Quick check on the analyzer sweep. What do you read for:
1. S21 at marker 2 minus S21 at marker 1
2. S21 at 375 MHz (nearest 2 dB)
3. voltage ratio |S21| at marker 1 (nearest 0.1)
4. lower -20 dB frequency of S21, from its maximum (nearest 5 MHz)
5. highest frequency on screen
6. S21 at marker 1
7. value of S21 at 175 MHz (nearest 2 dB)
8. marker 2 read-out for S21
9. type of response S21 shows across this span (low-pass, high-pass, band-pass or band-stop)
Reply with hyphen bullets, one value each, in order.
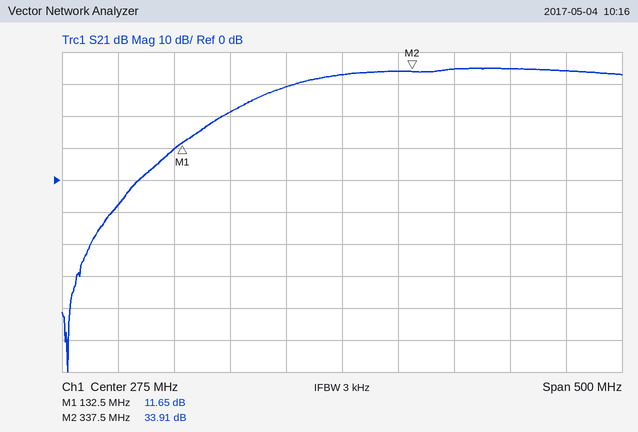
- 22.26 dB
- 34 dB
- 3.8
- 145 MHz
- 525 MHz
- 11.65 dB
- 22 dB
- 33.91 dB
- high-pass
